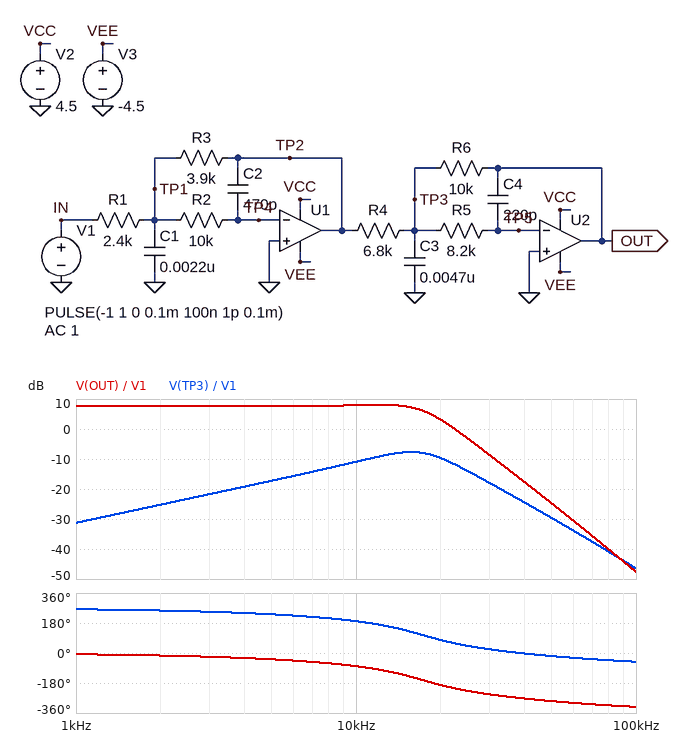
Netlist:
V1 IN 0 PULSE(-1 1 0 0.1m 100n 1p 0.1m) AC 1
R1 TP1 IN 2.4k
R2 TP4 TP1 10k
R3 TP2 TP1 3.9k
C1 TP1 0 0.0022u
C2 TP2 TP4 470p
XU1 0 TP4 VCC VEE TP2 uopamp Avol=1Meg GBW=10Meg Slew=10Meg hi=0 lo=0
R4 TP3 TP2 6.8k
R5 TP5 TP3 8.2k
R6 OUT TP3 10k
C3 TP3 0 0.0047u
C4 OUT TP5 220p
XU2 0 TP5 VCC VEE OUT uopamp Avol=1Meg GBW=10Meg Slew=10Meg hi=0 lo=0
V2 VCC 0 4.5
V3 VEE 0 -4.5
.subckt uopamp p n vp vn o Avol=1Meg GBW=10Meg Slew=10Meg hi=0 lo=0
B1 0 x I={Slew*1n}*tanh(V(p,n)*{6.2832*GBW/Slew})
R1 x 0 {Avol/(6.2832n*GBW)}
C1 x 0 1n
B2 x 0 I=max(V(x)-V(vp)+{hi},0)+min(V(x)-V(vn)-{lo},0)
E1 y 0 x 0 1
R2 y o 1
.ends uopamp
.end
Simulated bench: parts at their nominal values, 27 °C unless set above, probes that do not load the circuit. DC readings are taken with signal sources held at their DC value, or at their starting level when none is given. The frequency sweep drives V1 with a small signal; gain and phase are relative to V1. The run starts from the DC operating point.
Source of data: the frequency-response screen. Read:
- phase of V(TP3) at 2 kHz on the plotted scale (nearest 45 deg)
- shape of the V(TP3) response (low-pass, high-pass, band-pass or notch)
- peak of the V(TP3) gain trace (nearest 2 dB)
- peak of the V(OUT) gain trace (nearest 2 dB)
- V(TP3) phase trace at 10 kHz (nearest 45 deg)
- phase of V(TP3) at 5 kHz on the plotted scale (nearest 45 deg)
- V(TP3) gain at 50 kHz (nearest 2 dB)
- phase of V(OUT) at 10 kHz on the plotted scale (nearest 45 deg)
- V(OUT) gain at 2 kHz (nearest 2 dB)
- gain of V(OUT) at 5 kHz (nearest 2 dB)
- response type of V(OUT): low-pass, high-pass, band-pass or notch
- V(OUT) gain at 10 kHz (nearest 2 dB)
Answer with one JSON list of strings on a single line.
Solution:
["270 deg", "band-pass", "-8 dB", "8 dB", "180 deg", "225 deg", "-30 dB", "-90 deg", "8 dB", "8 dB", "low-pass", "8 dB"]
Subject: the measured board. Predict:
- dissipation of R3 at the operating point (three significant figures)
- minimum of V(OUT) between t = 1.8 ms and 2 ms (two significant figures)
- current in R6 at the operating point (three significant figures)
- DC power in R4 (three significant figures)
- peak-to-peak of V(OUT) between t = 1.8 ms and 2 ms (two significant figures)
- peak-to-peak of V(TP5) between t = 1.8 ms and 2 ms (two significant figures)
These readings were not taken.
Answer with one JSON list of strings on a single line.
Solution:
["677 µW", "-1.9 V", "239 µA", "388 µW", "3.5 V", "4.1 mV"]
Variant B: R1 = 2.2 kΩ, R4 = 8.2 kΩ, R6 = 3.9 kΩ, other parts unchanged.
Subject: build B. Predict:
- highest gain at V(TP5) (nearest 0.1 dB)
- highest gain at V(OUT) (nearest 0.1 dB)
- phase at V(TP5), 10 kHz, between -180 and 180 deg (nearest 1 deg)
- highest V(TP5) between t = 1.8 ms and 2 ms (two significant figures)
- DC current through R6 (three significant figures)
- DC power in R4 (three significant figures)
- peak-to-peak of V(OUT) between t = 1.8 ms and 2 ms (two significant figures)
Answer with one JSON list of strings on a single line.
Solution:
["-56.2 dB", "-1.5 dB", "-153 deg", "1.3 mV", "216 µA", "383 µW", "1.2 V"]
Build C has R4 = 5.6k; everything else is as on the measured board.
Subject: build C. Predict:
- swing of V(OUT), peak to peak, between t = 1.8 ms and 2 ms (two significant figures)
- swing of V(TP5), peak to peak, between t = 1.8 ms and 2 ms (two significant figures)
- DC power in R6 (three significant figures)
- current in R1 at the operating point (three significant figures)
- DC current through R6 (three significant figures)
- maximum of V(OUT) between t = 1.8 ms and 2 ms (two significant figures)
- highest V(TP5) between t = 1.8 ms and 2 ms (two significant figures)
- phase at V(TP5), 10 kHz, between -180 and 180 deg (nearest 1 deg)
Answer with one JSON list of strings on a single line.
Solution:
["4.1 V", "4.8 mV", "842 µW", "417 µA", "290 µA", "1.9 V", "3.1 mV", "-171 deg"]
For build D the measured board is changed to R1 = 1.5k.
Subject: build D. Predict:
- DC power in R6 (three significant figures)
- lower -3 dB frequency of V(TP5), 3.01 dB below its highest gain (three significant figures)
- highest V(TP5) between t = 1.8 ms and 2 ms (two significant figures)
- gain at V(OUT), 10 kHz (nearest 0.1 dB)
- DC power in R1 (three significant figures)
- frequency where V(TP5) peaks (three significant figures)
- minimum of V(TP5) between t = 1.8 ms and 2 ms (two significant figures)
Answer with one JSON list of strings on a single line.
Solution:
["1.46 mW", "9.47 kHz", "3.4 mV", "10.5 dB", "667 µW", "15.4 kHz", "-1.8 mV"]
